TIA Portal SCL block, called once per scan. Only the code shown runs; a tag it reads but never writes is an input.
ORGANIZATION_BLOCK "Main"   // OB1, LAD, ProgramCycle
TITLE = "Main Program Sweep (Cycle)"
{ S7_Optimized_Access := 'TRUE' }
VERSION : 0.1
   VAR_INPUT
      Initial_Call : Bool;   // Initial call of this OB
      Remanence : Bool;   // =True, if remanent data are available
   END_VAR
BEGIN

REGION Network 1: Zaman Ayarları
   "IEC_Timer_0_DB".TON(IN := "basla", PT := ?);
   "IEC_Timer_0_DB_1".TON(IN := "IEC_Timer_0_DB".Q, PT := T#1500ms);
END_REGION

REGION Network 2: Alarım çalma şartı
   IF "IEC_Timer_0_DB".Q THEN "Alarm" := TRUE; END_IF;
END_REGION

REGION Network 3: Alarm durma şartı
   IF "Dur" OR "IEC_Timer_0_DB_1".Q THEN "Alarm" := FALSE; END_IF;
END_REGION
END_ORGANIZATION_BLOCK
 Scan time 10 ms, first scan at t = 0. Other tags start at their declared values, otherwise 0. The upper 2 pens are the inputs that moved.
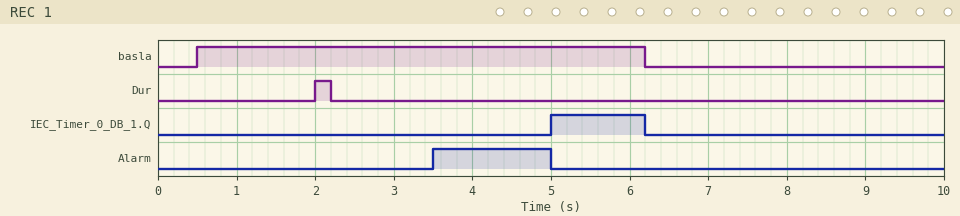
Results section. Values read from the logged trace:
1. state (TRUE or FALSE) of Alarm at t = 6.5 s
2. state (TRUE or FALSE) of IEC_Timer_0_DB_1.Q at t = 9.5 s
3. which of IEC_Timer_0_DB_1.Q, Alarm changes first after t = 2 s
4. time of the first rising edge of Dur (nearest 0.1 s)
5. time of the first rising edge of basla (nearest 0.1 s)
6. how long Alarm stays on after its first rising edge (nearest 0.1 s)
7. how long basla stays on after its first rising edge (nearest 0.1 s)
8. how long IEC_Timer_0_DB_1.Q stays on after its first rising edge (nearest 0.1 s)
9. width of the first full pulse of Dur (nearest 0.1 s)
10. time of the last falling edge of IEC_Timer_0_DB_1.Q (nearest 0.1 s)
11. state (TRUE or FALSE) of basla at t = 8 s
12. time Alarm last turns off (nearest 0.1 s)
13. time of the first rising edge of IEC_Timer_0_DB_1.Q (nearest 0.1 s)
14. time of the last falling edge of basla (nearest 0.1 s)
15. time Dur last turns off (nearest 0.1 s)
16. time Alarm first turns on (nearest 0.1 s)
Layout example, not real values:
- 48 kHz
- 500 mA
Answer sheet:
- FALSE
- FALSE
- Alarm
- 2.0 s
- 0.5 s
- 1.5 s
- 5.7 s
- 1.2 s
- 0.2 s
- 6.2 s
- FALSE
- 5.0 s
- 5.0 s
- 6.2 s
- 2.2 s
- 3.5 s
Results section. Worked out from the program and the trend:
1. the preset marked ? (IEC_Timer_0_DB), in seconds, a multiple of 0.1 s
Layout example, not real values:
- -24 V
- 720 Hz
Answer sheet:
- 3.0 s
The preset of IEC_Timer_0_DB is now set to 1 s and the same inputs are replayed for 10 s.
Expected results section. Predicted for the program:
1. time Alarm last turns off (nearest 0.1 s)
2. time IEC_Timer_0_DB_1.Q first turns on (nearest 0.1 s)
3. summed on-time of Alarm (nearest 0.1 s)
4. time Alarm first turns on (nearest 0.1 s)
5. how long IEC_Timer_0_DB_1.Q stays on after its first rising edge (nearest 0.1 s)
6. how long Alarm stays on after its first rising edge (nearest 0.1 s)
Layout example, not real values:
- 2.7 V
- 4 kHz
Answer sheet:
- 3.0 s
- 3.0 s
- 1.3 s
- 1.5 s
- 3.2 s
- 0.5 s
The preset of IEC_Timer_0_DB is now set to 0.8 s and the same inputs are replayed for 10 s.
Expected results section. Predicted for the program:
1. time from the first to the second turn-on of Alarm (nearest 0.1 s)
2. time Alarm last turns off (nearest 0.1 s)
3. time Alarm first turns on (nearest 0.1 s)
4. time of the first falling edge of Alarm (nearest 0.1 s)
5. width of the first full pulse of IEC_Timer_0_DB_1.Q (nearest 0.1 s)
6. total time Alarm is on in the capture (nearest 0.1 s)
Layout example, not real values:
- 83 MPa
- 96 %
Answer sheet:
- 0.9 s
- 2.8 s
- 1.3 s
- 2.0 s
- 3.4 s
- 1.3 s
